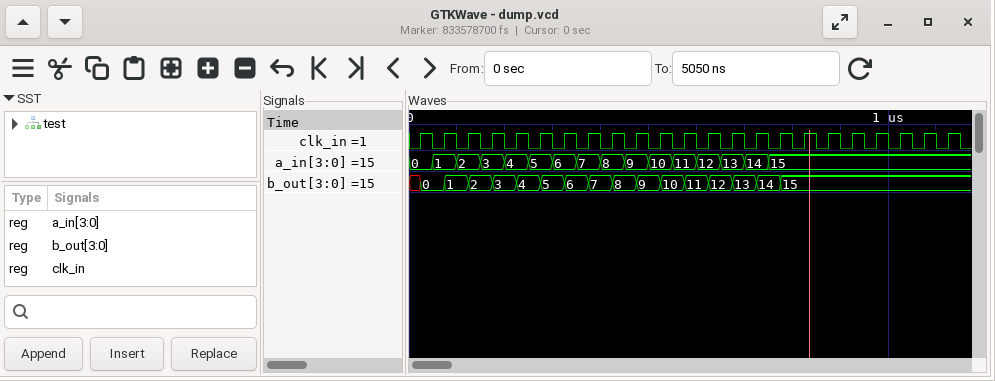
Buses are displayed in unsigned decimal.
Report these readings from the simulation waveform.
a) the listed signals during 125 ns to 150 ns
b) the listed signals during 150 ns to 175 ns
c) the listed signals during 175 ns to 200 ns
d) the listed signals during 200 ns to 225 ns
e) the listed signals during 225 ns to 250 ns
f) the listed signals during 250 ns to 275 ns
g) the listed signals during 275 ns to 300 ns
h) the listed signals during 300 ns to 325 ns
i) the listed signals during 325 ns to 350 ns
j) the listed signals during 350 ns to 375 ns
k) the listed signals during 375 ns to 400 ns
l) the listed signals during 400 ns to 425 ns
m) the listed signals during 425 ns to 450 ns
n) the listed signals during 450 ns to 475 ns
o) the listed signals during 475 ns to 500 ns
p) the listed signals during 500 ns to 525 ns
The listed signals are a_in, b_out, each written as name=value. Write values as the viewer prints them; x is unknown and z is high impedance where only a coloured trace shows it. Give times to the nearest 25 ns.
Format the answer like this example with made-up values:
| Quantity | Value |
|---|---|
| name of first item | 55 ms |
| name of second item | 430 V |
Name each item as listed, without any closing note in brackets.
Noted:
| Quantity | Value |
|---|---|
| the listed signals during 125 ns to 150 ns | a_in=2, b_out=2 |
| the listed signals during 150 ns to 175 ns | a_in=3, b_out=2 |
| the listed signals during 175 ns to 200 ns | a_in=3, b_out=3 |
| the listed signals during 200 ns to 225 ns | a_in=4, b_out=3 |
| the listed signals during 225 ns to 250 ns | a_in=4, b_out=4 |
| the listed signals during 250 ns to 275 ns | a_in=5, b_out=4 |
| the listed signals during 275 ns to 300 ns | a_in=5, b_out=5 |
| the listed signals during 300 ns to 325 ns | a_in=6, b_out=5 |
| the listed signals during 325 ns to 350 ns | a_in=6, b_out=6 |
| the listed signals during 350 ns to 375 ns | a_in=7, b_out=6 |
| the listed signals during 375 ns to 400 ns | a_in=7, b_out=7 |
| the listed signals during 400 ns to 425 ns | a_in=8, b_out=7 |
| the listed signals during 425 ns to 450 ns | a_in=8, b_out=8 |
| the listed signals during 450 ns to 475 ns | a_in=9, b_out=8 |
| the listed signals during 475 ns to 500 ns | a_in=9, b_out=9 |
| the listed signals during 500 ns to 525 ns | a_in=10, b_out=9 |
